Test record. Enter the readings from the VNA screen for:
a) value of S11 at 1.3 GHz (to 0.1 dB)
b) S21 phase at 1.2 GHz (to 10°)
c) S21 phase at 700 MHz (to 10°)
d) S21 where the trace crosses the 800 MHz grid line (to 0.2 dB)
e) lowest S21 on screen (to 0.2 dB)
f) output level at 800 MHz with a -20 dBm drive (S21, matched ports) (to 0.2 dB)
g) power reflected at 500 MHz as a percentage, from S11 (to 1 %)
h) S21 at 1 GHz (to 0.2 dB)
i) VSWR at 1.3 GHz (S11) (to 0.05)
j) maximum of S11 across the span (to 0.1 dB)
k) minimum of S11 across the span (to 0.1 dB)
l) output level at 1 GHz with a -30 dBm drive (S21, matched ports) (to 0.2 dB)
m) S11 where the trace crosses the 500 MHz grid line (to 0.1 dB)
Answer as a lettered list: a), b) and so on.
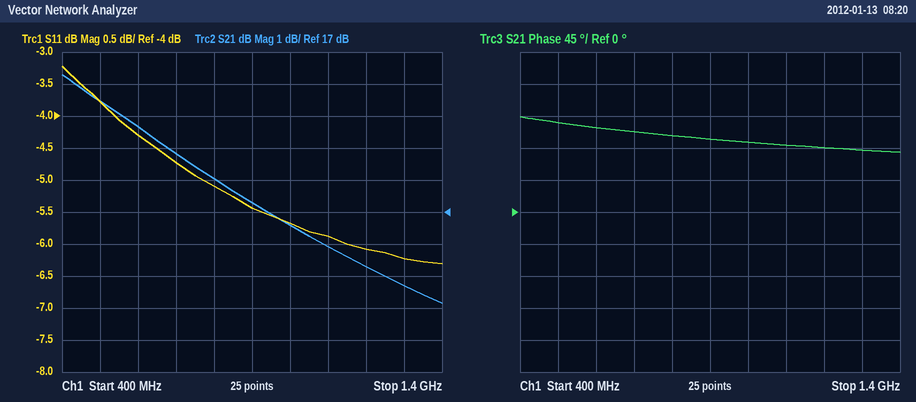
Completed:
a) -6.2 dB
b) 90°
c) 110°
d) 18.0 dB
e) 14.2 dB
f) -2.0 dBm
g) 42 %
h) 16.6 dB
i) 2.90
j) -3.2 dB
k) -6.3 dB
l) -13.4 dBm
m) -3.8 dB
